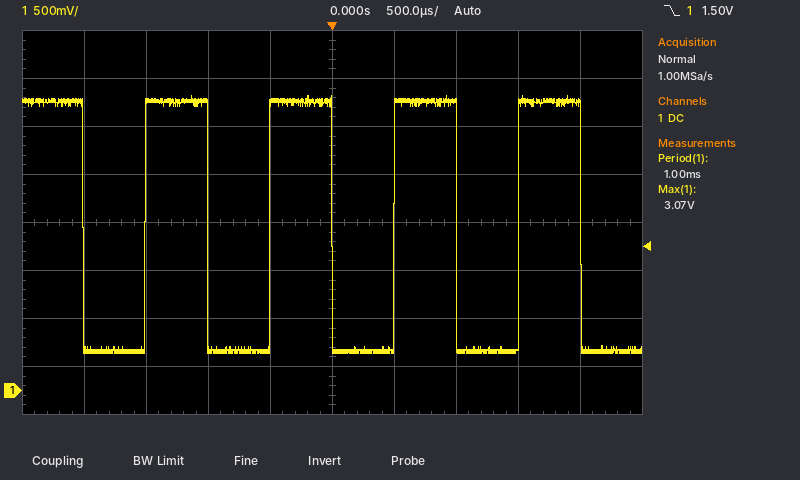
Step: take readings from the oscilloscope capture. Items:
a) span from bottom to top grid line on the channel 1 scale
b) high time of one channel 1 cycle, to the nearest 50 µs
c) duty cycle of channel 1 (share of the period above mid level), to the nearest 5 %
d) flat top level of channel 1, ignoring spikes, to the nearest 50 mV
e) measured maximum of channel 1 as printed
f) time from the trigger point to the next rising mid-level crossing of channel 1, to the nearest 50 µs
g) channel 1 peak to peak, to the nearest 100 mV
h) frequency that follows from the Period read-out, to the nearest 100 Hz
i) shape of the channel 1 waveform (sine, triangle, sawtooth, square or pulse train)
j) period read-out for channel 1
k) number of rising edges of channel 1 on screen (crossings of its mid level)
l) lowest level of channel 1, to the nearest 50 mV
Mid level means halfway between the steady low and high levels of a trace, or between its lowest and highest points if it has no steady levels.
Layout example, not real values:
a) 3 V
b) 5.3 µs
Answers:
a) 4 V
b) 500 µs
c) 50 %
d) 3.00 V
e) 3.07 V
f) 500 µs
g) 2.70 V
h) 1.0 kHz
i) square
j) 1.00 ms
k) 4
l) 400 mV
